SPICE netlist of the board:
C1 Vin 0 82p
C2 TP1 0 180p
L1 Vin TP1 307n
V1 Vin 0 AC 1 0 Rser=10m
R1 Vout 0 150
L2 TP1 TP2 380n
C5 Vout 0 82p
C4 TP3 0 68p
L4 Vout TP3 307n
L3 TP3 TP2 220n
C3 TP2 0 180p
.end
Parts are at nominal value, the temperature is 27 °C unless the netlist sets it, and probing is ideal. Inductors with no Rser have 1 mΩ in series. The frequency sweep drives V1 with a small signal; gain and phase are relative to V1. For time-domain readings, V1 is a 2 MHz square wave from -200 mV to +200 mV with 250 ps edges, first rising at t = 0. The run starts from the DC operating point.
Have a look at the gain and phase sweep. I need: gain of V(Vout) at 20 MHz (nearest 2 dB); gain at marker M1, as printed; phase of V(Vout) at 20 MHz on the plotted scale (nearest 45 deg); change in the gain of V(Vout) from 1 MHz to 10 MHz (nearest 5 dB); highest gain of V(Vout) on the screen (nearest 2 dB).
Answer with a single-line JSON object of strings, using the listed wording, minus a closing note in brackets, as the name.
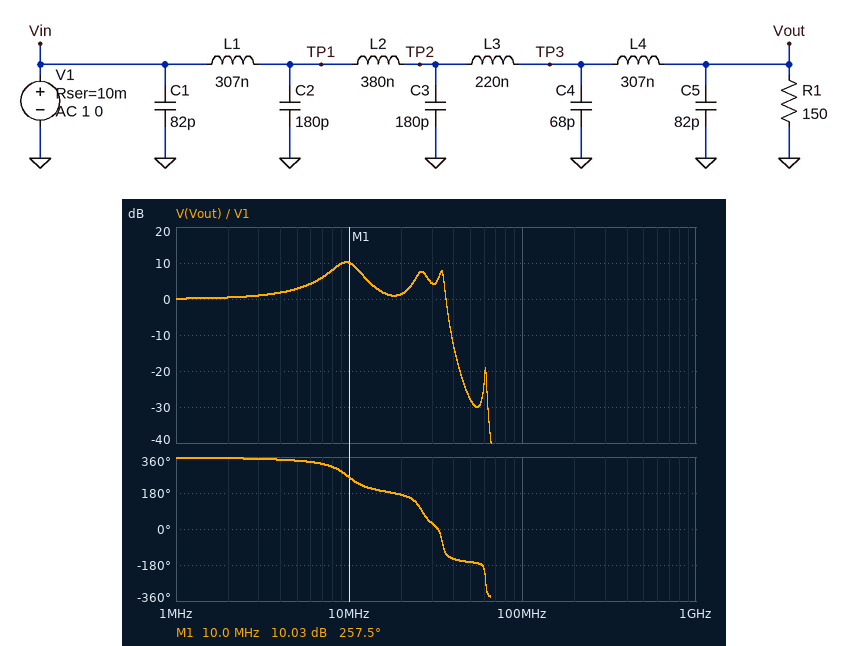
{"gain of V(Vout) at 20 MHz": "2 dB", "gain at marker M1, as printed": "10.03 dB", "phase of V(Vout) at 20 MHz on the plotted scale": "180 deg", "change in the gain of V(Vout) from 1 MHz to 10 MHz": "10 dB", "highest gain of V(Vout) on the screen": "10 dB"}
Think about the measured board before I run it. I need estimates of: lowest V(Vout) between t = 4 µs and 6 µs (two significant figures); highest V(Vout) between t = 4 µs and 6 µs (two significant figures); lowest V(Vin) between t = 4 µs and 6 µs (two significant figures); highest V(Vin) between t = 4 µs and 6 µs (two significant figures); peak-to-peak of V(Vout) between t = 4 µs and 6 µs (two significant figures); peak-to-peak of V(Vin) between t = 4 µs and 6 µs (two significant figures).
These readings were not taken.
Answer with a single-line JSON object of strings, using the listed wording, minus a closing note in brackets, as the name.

{"lowest V(Vout) between t = 4 µs and 6 µs": "-560 mV", "highest V(Vout) between t = 4 µs and 6 µs": "560 mV", "lowest V(Vin) between t = 4 µs and 6 µs": "-200 mV", "highest V(Vin) between t = 4 µs and 6 µs": "200 mV", "peak-to-peak of V(Vout) between t = 4 µs and 6 µs": "1.1 V", "peak-to-peak of V(Vin) between t = 4 µs and 6 µs": "400 mV"}
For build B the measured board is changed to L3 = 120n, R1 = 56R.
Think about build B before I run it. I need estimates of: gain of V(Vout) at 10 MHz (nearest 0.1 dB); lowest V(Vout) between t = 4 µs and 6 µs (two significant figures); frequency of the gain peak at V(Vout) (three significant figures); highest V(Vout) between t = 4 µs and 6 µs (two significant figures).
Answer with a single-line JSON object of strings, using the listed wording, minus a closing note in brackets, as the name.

{"gain of V(Vout) at 10 MHz": "2.1 dB", "lowest V(Vout) between t = 4 µs and 6 µs": "-320 mV", "frequency of the gain peak at V(Vout)": "32.3 MHz", "highest V(Vout) between t = 4 µs and 6 µs": "320 mV"}
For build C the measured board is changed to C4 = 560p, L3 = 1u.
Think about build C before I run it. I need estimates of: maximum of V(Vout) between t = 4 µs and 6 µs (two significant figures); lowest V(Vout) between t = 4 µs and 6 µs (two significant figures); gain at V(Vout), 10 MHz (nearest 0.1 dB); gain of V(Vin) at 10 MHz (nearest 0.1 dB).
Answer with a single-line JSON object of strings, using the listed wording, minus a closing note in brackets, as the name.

{"maximum of V(Vout) between t = 4 µs and 6 µs": "450 mV", "lowest V(Vout) between t = 4 µs and 6 µs": "-450 mV", "gain at V(Vout), 10 MHz": "-5.6 dB", "gain of V(Vin) at 10 MHz": "0 dB"}
